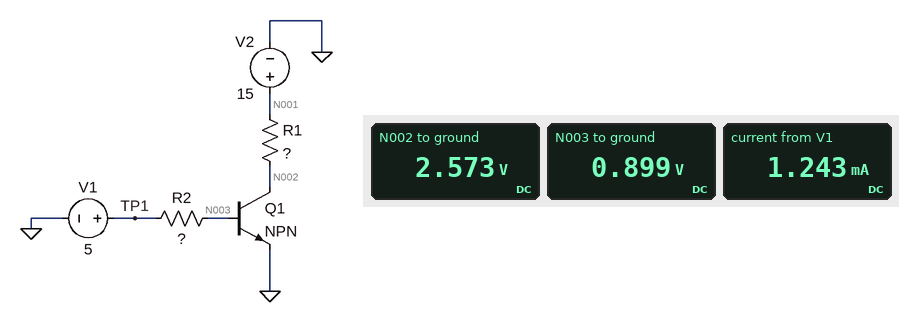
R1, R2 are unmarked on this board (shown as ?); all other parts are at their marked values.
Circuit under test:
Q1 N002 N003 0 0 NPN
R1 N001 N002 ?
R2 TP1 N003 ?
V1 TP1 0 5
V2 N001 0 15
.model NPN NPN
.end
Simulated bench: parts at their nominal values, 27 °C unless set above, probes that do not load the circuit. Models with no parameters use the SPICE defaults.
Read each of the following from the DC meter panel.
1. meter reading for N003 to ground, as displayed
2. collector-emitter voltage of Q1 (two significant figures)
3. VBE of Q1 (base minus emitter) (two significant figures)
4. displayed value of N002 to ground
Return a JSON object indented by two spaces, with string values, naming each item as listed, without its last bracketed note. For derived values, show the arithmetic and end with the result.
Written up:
{
  "meter reading for N003 to ground, as displayed": "0.899 V",
  "collector-emitter voltage of Q1": "2.573 V = 2.6 V",
  "VBE of Q1 (base minus emitter)": "899 mV = 900 mV",
  "displayed value of N002 to ground": "2.573 V"
}
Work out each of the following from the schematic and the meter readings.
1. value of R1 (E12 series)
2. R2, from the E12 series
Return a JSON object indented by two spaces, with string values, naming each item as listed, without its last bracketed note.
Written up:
{
  "value of R1": "100 Ω",
  "R2, from the E12 series": "3.3 kΩ"
}
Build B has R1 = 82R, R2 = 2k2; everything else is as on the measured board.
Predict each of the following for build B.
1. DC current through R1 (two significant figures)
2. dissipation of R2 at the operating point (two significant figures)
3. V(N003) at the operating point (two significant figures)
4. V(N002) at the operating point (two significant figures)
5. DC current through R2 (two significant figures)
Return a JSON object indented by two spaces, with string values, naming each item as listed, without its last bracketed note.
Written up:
{
  "DC current through R1": "180 mA",
  "dissipation of R2 at the operating point": "7.6 mW",
  "V(N003) at the operating point": "910 mV",
  "V(N002) at the operating point": "210 mV",
  "DC current through R2": "1.9 mA"
}
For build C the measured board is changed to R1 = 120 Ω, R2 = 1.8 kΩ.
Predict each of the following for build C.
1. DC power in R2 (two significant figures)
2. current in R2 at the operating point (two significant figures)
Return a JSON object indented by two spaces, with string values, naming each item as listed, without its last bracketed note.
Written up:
{
  "DC power in R2": "9.3 mW",
  "current in R2 at the operating point": "2.3 mA"
}
